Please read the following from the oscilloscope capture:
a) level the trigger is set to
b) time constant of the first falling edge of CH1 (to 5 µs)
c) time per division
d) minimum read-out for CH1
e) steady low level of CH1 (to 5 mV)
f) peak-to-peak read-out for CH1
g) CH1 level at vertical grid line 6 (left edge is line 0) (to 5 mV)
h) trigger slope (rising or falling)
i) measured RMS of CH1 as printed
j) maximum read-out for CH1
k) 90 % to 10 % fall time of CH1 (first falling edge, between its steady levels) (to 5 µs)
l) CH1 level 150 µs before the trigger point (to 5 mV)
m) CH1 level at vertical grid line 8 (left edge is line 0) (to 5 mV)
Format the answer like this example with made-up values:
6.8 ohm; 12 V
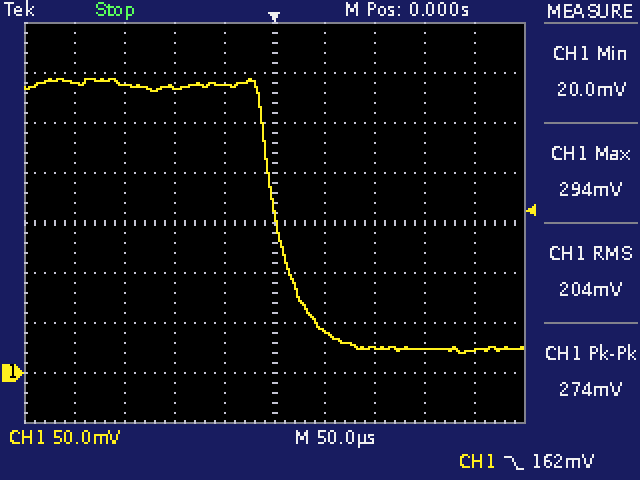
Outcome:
162 mV; 25 µs; 50 µs; 20.0 mV; 25 mV; 274 mV; 40 mV; falling; 204 mV; 294 mV; 55 µs; 290 mV; 25 mV
